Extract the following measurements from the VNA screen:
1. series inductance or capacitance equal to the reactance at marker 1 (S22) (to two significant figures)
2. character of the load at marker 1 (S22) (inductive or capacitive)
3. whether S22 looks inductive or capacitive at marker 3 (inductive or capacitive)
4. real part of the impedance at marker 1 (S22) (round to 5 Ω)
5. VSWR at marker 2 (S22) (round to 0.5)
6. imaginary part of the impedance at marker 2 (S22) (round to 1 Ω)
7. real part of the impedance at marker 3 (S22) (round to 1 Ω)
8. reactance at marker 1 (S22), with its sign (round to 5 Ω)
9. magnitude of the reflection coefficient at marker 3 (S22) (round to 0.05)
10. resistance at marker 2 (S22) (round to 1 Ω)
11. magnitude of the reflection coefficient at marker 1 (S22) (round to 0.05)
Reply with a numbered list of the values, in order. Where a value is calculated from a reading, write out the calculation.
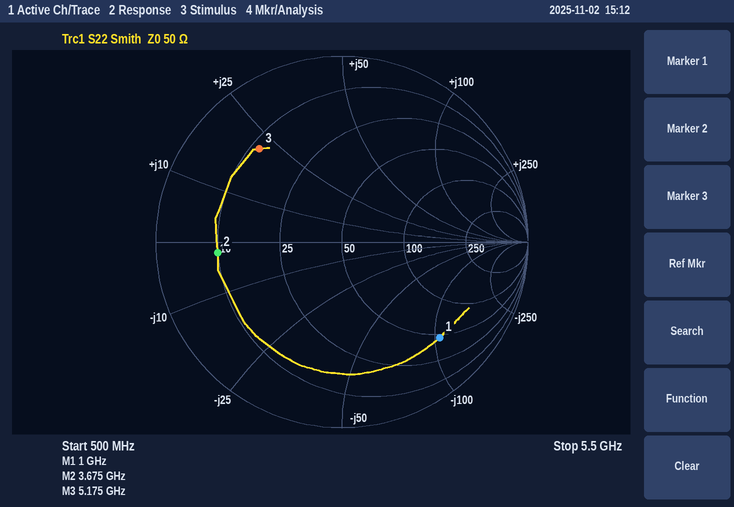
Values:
1. C = 1/(2π × 1 GHz × 105 Ω) ≈ 1.5 pF
2. capacitive
3. inductive
4. 45 Ω
5. 5.0
6. -2 Ω
7. 12 Ω
8. -105 Ω
9. 0.65
10. 10 Ω
11. 0.75
